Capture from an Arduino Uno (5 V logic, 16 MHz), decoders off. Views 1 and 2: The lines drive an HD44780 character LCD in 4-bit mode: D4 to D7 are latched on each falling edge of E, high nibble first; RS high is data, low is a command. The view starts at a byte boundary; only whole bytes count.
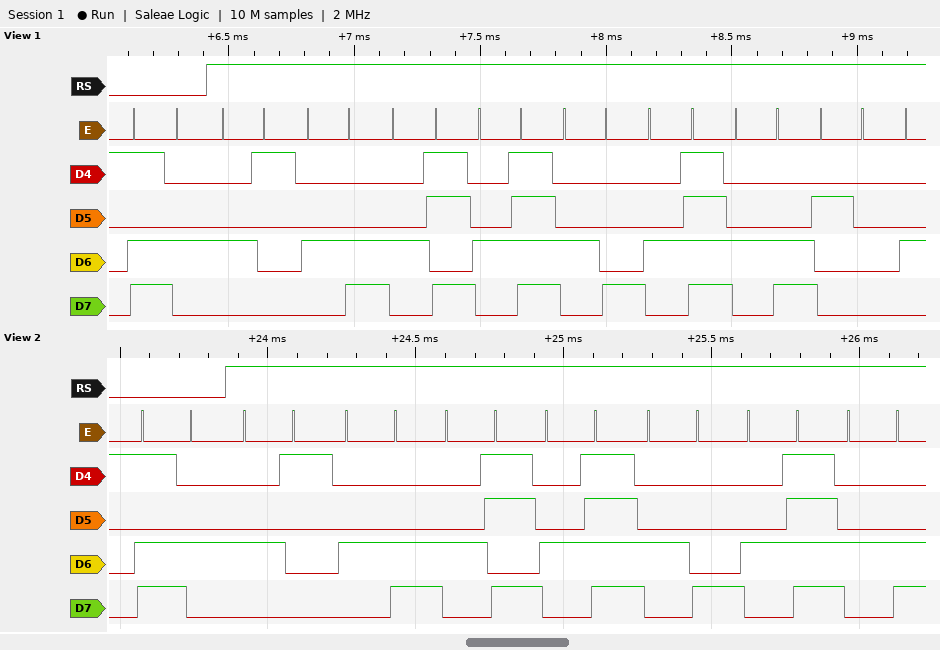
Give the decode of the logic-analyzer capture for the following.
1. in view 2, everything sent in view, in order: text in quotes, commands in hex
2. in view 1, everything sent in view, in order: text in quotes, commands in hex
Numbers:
0xD4 "ALKOHOL"
0xD4 "ALKOHOL "
